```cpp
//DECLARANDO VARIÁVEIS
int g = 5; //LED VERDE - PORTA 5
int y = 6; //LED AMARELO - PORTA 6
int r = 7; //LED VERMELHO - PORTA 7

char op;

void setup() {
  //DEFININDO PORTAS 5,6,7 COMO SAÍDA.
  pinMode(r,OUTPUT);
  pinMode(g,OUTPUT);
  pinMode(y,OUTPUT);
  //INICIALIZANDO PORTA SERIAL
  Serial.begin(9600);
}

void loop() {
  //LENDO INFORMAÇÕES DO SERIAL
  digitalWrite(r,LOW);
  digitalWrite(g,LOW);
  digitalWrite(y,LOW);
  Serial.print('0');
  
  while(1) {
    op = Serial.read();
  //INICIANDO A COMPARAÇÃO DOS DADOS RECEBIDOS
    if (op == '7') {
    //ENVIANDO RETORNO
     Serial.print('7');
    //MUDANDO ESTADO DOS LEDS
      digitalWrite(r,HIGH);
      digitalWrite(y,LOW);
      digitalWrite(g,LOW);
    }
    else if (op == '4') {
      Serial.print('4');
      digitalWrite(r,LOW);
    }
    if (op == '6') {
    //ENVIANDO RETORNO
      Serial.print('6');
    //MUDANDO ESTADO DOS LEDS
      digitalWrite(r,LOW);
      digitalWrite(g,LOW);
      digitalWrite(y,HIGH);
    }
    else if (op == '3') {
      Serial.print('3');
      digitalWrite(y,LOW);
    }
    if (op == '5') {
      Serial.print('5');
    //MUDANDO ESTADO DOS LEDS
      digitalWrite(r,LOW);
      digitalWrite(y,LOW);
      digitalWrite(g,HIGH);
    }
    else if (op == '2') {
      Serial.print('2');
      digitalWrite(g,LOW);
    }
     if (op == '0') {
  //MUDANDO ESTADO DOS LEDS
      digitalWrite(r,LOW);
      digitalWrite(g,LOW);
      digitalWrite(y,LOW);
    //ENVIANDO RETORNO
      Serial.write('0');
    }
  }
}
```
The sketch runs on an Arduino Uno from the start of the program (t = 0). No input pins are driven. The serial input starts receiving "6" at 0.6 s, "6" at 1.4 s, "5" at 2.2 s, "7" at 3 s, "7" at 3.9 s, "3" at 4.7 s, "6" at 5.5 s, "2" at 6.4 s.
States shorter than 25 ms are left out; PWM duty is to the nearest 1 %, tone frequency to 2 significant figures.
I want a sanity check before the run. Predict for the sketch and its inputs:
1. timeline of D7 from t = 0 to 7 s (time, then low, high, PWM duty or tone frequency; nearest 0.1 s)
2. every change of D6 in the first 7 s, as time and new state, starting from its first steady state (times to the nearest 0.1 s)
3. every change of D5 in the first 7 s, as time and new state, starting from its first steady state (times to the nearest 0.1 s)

0 s low; 3 s high; 5.5 s low
0 s low; 0.6 s high; 2.2 s low; 5.5 s high
0 s low; 2.2 s high; 3 s low
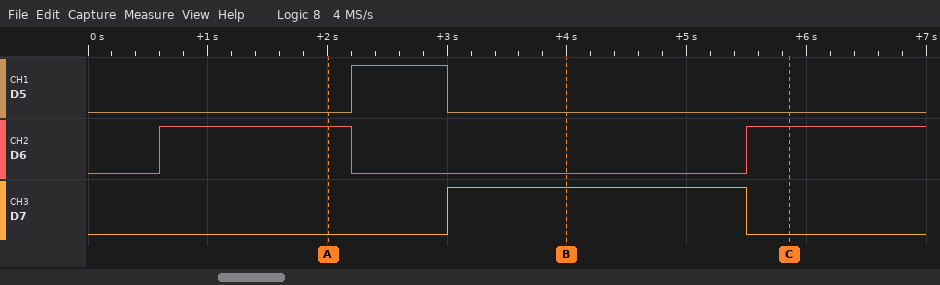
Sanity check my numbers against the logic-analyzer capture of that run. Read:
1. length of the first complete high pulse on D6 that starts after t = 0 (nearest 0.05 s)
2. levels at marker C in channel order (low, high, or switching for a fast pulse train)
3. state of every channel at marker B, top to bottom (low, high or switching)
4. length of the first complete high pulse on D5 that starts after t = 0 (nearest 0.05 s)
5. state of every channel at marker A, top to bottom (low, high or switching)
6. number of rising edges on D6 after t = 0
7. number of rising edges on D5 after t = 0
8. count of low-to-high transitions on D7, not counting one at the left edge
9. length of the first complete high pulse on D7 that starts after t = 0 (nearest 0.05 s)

1.60 s
D5 low, D6 high, D7 low
D5 low, D6 low, D7 high
0.80 s
D5 low, D6 high, D7 low
2
1
1
2.50 s
